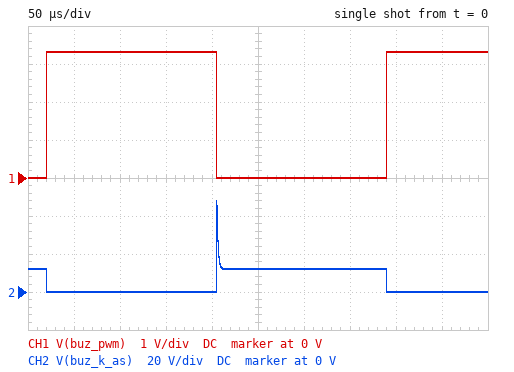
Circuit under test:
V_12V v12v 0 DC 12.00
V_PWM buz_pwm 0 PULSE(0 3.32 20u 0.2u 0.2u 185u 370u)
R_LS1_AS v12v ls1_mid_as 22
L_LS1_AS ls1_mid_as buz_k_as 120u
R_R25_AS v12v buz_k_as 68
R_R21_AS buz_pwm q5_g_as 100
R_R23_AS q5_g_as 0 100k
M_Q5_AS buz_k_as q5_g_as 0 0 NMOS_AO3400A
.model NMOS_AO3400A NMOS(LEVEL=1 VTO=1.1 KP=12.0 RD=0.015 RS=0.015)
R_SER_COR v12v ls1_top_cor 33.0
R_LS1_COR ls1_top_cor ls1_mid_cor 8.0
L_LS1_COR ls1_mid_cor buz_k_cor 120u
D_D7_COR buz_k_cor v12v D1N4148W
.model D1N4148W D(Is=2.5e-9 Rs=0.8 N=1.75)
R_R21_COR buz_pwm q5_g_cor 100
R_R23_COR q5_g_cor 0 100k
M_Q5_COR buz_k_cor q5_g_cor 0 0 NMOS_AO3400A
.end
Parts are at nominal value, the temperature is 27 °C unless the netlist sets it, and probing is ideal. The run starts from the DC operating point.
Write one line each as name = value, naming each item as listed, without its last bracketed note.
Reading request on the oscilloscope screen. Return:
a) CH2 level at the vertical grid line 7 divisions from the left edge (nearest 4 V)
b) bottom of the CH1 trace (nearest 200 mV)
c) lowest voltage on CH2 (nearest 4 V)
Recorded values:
CH2 level at the vertical grid line 7 divisions from the left edge = 12 V
bottom of the CH1 trace = 0 V
lowest voltage on CH2 = 0 V
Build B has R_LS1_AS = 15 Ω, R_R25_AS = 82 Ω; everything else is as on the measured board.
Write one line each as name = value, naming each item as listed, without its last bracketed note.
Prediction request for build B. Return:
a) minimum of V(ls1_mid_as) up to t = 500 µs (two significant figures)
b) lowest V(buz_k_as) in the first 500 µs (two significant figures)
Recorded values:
minimum of V(ls1_mid_as) up to t = 500 µs = 64 mV
lowest V(buz_k_as) in the first 500 µs = 11 mV
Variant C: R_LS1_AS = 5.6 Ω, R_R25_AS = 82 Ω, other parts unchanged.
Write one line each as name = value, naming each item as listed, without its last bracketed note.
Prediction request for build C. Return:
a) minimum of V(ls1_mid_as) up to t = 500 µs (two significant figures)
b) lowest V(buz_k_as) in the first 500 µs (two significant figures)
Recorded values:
minimum of V(ls1_mid_as) up to t = 500 µs = 160 mV
lowest V(buz_k_as) in the first 500 µs = 11 mV
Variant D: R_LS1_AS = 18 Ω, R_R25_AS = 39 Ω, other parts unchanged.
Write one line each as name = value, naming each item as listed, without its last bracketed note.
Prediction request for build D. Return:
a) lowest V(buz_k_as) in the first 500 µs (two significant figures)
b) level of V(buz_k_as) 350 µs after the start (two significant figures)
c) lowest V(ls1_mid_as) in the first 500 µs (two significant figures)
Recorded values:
lowest V(buz_k_as) in the first 500 µs = 22 mV
level of V(buz_k_as) 350 µs after the start = 12 V
lowest V(ls1_mid_as) in the first 500 µs = 66 mV
